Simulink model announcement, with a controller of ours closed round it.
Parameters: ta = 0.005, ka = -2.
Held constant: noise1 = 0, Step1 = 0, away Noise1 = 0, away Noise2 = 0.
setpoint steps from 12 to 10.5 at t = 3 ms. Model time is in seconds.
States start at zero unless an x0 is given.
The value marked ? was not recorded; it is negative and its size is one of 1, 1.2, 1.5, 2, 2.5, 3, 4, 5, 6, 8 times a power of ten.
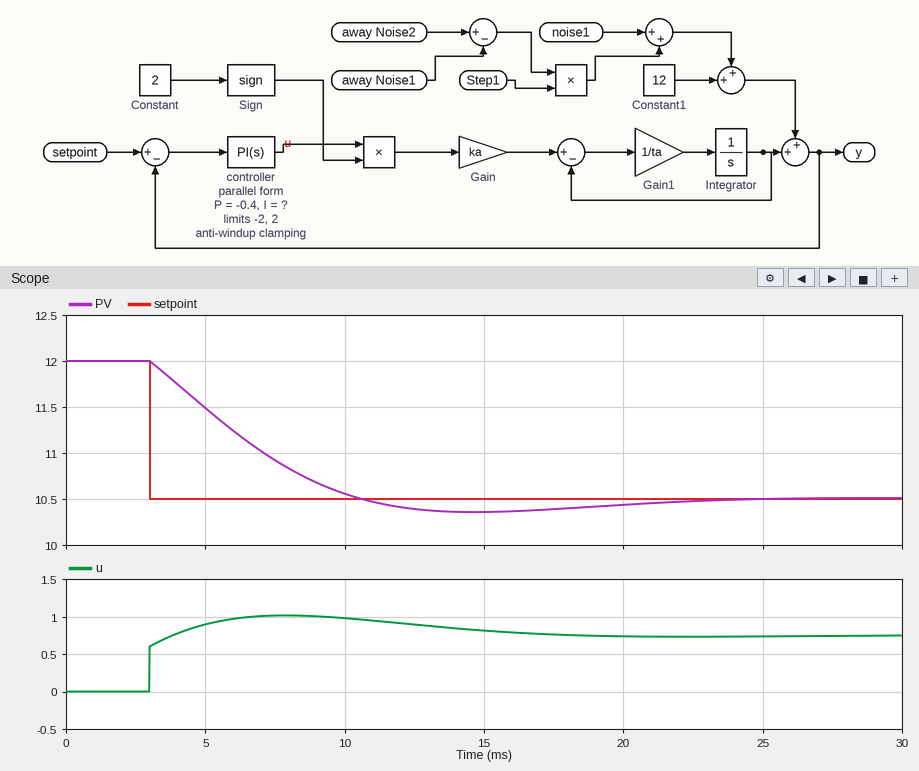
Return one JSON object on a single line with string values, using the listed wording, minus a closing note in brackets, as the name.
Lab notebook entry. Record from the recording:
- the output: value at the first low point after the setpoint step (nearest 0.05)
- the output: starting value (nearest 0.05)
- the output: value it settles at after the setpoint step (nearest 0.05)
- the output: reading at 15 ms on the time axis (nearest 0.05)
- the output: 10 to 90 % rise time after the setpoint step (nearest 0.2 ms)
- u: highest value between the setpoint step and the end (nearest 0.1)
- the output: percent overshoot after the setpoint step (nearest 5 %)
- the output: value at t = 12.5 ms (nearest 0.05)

{"the output: value at the first low point after the setpoint step": "10.35", "the output: starting value": "12.00", "the output: value it settles at after the setpoint step": "10.50", "the output: reading at 15 ms on the time axis": "10.35", "the output: 10 to 90 % rise time after the setpoint step": "5.6 ms", "u: highest value between the setpoint step and the end": "1.0", "the output: percent overshoot after the setpoint step": "10 %", "the output: value at t = 12.5 ms": "10.40"}
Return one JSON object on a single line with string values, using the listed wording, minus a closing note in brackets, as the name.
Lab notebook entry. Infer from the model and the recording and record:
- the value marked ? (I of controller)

{"the value marked ?": "-200"}
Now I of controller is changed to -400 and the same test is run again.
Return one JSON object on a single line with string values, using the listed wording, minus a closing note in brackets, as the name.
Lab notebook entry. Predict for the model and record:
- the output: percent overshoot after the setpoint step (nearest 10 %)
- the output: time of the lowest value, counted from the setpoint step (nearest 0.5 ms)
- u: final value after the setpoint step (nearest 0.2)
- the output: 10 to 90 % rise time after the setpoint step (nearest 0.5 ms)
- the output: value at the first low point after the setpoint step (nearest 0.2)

{"the output: percent overshoot after the setpoint step": "20 %", "the output: time of the lowest value, counted from the setpoint step": "7.5 ms", "u: final value after the setpoint step": "0.8", "the output: 10 to 90 % rise time after the setpoint step": "3.5 ms", "the output: value at the first low point after the setpoint step": "10.2"}
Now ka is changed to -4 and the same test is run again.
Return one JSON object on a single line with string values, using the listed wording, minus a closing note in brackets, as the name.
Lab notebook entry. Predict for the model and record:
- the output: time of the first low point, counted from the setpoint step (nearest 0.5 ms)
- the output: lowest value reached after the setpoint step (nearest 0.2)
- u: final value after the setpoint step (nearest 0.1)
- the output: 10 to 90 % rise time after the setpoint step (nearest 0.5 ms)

{"the output: time of the first low point, counted from the setpoint step": "7.5 ms", "the output: lowest value reached after the setpoint step": "10.4", "u: final value after the setpoint step": "0.4", "the output: 10 to 90 % rise time after the setpoint step": "3.5 ms"}
